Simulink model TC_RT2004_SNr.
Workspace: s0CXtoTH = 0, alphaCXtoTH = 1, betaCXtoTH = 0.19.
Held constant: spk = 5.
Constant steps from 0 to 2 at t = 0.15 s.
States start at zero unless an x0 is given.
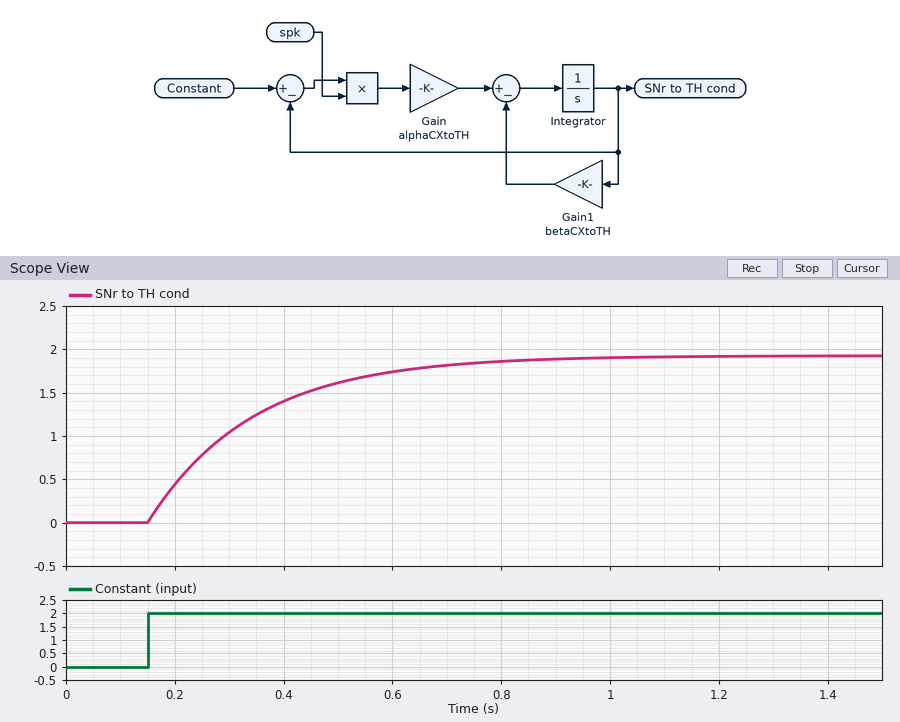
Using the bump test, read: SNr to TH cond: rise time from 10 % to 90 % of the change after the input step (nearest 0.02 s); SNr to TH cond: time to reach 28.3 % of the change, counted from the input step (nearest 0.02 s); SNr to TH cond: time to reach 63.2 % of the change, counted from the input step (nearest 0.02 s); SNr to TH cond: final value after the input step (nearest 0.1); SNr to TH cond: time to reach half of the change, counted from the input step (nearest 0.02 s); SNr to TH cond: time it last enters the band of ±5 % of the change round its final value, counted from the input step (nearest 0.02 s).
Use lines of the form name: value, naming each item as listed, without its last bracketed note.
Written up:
SNr to TH cond: rise time from 10 % to 90 % of the change after the input step: 0.42 s
SNr to TH cond: time to reach 28.3 % of the change, counted from the input step: 0.06 s
SNr to TH cond: time to reach 63.2 % of the change, counted from the input step: 0.20 s
SNr to TH cond: final value after the input step: 1.9
SNr to TH cond: time to reach half of the change, counted from the input step: 0.14 s
SNr to TH cond: time it last enters the band of ±5 % of the change round its final value, counted from the input step: 0.58 s
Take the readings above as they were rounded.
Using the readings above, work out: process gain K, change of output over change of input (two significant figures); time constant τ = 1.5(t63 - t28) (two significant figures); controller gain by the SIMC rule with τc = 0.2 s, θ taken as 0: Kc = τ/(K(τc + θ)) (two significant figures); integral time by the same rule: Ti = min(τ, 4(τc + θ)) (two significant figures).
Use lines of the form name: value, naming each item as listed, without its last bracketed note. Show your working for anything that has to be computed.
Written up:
process gain K, change of output over change of input: (1.9 - 0) / 2 = 0.95
time constant τ = 1.5(t63 - t28): 1.5 × (0.2 - 0.06) = 0.21 s
controller gain by the SIMC rule with τc = 0.2 s, θ taken as 0: Kc = τ/(K(τc + θ)): 0.21 / (0.95 × (0.2 + 0)) = 1.1
integral time by the same rule: Ti = min(τ, 4(τc + θ)): min(0.21, 4 × (0.2 + 0)) = 0.21 s
